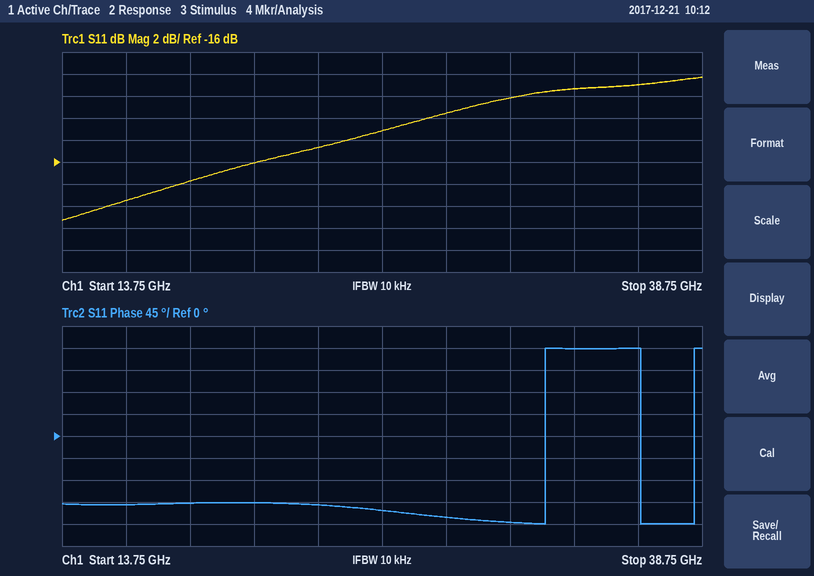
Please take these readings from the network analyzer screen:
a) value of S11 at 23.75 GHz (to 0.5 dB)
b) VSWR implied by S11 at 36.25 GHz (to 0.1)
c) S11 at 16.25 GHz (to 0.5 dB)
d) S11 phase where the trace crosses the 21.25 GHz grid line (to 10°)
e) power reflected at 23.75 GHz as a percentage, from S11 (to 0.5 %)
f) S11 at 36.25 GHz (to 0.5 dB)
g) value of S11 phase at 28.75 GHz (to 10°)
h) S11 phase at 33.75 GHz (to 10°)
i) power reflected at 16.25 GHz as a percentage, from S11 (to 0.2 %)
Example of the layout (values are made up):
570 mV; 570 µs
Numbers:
-14.5 dB; 2.1; -19.5 dB; -140°; 3.5 %; -9.0 dB; -170°; 180°; 1.2 %
